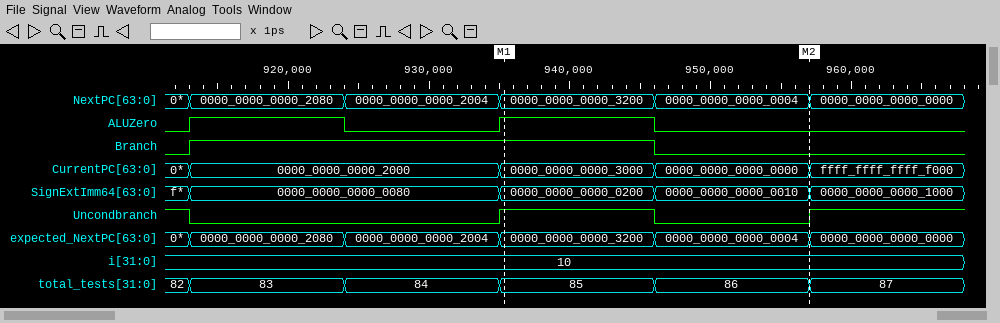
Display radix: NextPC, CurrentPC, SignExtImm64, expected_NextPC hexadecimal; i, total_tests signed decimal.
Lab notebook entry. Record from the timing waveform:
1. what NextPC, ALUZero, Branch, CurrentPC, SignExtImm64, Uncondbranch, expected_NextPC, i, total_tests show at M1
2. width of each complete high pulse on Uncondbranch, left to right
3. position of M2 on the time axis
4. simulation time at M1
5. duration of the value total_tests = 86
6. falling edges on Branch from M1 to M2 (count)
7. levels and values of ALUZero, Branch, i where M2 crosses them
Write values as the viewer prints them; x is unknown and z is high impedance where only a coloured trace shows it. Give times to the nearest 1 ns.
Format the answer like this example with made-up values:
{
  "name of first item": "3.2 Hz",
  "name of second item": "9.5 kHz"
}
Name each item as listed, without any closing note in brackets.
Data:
{
  "what NextPC, ALUZero, Branch, CurrentPC, SignExtImm64, Uncondbranch, expected_NextPC, i, total_tests show at M1": "NextPC=0000_0000_0000_3200, ALUZero=1, Branch=1, CurrentPC=0000_0000_0000_3000, SignExtImm64=0000_0000_0000_0200, Uncondbranch=1, expected_NextPC=0000_0000_0000_3200, i=10, total_tests=85",
  "width of each complete high pulse on Uncondbranch, left to right": "11 ns",
  "position of M2 on the time axis": "957 ns",
  "simulation time at M1": "935 ns",
  "duration of the value total_tests = 86": "11 ns",
  "falling edges on Branch from M1 to M2": "1",
  "levels and values of ALUZero, Branch, i where M2 crosses them": "ALUZero=0, Branch=0, i=10"
}
